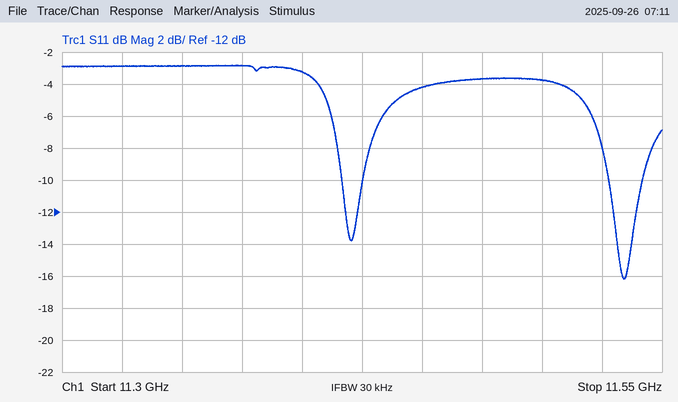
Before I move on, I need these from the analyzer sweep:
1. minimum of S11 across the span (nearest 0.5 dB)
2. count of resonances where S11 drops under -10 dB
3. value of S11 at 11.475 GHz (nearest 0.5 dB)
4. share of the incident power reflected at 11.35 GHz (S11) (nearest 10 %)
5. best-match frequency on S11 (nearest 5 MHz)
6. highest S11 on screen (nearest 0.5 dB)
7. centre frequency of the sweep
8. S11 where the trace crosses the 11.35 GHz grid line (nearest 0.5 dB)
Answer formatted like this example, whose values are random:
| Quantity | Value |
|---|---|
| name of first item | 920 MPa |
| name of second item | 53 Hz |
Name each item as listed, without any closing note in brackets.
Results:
| Quantity | Value |
|---|---|
| minimum of S11 across the span | -16.0 dB |
| count of resonances where S11 drops under -10 dB | 2 |
| value of S11 at 11.475 GHz | -3.5 dB |
| share of the incident power reflected at 11.35 GHz (S11) | 50 % |
| best-match frequency on S11 | 11.535 GHz |
| highest S11 on screen | -3.0 dB |
| centre frequency of the sweep | 11.425 GHz |
| S11 where the trace crosses the 11.35 GHz grid line | -3.0 dB |
